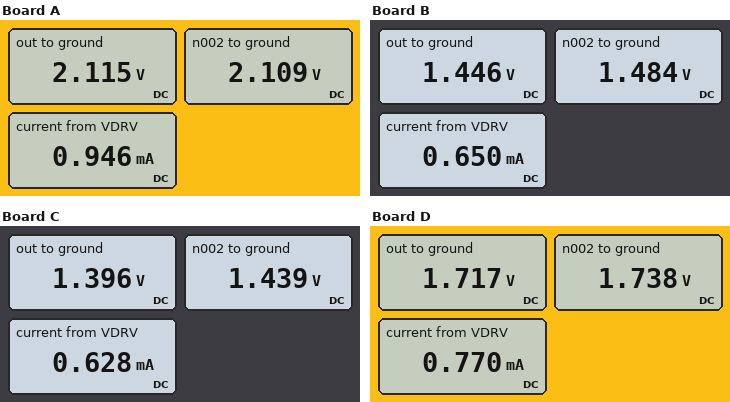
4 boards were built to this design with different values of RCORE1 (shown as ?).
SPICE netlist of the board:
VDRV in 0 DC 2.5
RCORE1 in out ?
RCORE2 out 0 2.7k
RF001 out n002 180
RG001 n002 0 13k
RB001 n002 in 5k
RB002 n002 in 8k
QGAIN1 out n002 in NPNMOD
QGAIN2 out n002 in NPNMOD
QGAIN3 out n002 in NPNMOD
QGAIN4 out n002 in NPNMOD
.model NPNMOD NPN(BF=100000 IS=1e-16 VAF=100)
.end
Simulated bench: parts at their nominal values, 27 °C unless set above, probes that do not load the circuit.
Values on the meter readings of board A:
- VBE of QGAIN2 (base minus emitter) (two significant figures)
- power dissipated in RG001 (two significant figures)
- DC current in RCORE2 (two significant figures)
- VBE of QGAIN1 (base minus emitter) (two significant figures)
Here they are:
-390 mV
340 µW
780 µA
-390 mV
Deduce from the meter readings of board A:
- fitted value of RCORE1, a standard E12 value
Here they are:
470 Ω
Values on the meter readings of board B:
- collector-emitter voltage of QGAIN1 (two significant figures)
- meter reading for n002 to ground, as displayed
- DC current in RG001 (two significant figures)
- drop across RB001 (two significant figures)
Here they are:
-1.1 V
1.484 V
110 µA
1.0 V
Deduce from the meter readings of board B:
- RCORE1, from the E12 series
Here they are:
3.3 kΩ
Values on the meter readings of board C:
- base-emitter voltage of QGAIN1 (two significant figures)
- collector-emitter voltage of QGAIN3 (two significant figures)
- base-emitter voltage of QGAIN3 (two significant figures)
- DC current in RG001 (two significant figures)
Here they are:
-1.1 V
-1.1 V
-1.1 V
110 µA
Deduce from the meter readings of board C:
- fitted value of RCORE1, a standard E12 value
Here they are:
3.9 kΩ
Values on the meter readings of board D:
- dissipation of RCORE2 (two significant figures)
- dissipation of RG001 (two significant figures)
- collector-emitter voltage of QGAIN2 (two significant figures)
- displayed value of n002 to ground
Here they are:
1.1 mW
230 µW
-780 mV
1.738 V
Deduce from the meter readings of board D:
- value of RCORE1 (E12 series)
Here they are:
1.5 kΩ
